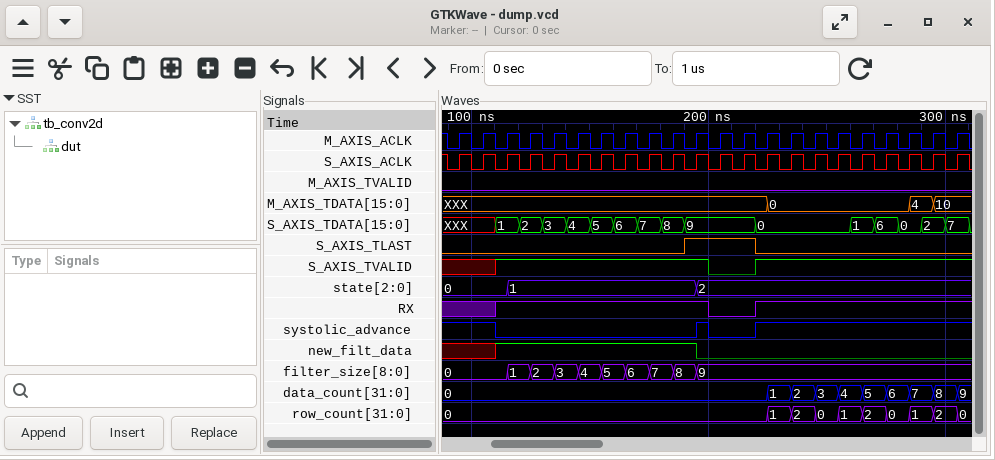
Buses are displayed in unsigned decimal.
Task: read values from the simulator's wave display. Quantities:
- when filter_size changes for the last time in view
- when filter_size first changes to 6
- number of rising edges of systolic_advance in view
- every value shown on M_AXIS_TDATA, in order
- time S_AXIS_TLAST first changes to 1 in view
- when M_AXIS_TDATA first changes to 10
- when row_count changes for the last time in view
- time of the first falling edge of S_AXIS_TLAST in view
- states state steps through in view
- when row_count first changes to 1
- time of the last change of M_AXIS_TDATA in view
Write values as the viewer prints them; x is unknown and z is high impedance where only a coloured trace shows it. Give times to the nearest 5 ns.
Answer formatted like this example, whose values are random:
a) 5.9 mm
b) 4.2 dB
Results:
a) 195 ns
b) 165 ns
c) 2
d) XXX, 0, 4, 10
e) 190 ns
f) 295 ns
g) 305 ns
h) 220 ns
i) 0, 1, 2
j) 225 ns
k) 295 ns
